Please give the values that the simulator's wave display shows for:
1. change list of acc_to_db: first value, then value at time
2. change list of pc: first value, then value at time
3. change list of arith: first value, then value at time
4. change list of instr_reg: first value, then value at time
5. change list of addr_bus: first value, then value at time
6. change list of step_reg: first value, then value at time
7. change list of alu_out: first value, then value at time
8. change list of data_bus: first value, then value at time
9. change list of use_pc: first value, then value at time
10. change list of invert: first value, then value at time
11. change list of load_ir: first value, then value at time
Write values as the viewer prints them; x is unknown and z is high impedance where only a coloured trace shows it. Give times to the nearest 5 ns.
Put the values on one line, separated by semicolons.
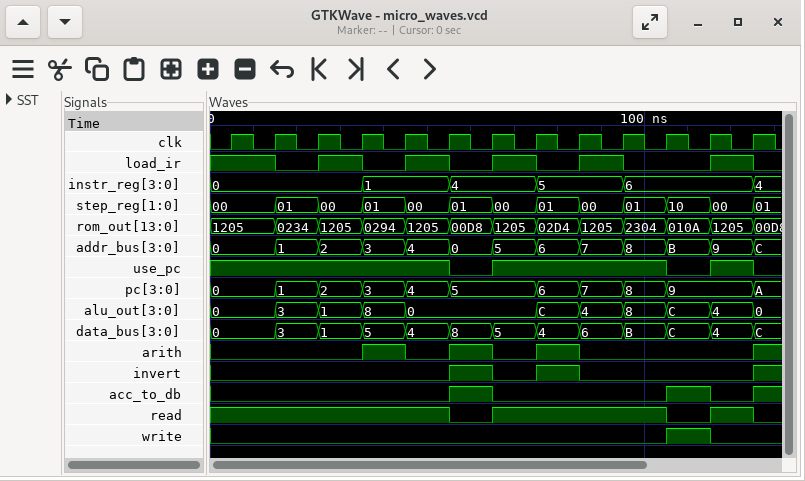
0, 1 at 55 ns, 0 at 65 ns, 1 at 105 ns, 0 at 115 ns, 1 at 125 ns; 0, 1 at 15 ns, 2 at 25 ns, 3 at 35 ns, 4 at 45 ns, 5 at 55 ns, 6 at 75 ns, 7 at 85 ns, 8 at 95 ns, 9 at 105 ns, A at 125 ns; 0, 1 at 35 ns, 0 at 45 ns, 1 at 55 ns, 0 at 65 ns, 1 at 75 ns, 0 at 85 ns, 1 at 125 ns; 0, 1 at 35 ns, 4 at 55 ns, 5 at 75 ns, 6 at 95 ns, 4 at 125 ns; 0, 1 at 15 ns, 2 at 25 ns, 3 at 35 ns, 4 at 45 ns, 0 at 55 ns, 5 at 65 ns, 6 at 75 ns, 7 at 85 ns, 8 at 95 ns, B at 105 ns, 9 at 115 ns, C at 125 ns; 00, 01 at 15 ns, 00 at 25 ns, 01 at 35 ns, 00 at 45 ns, 01 at 55 ns, 00 at 65 ns, 01 at 75 ns, 00 at 85 ns, 01 at 95 ns, 10 at 105 ns, 00 at 115 ns, 01 at 125 ns; 0, 3 at 15 ns, 1 at 25 ns, 8 at 35 ns, 0 at 45 ns, C at 75 ns, 4 at 85 ns, 8 at 95 ns, C at 105 ns, 4 at 115 ns, 0 at 125 ns; 0, 3 at 15 ns, 1 at 25 ns, 5 at 35 ns, 4 at 45 ns, 8 at 55 ns, 5 at 65 ns, 4 at 75 ns, 6 at 85 ns, B at 95 ns, C at 105 ns, 4 at 115 ns, C at 125 ns; 1, 0 at 55 ns, 1 at 65 ns, 0 at 105 ns, 1 at 115 ns, 0 at 125 ns; 0, 1 at 55 ns, 0 at 65 ns, 1 at 75 ns, 0 at 85 ns, 1 at 125 ns; 1, 0 at 15 ns, 1 at 25 ns, 0 at 35 ns, 1 at 45 ns, 0 at 55 ns, 1 at 65 ns, 0 at 75 ns, 1 at 85 ns, 0 at 95 ns, 1 at 115 ns, 0 at 125 ns
